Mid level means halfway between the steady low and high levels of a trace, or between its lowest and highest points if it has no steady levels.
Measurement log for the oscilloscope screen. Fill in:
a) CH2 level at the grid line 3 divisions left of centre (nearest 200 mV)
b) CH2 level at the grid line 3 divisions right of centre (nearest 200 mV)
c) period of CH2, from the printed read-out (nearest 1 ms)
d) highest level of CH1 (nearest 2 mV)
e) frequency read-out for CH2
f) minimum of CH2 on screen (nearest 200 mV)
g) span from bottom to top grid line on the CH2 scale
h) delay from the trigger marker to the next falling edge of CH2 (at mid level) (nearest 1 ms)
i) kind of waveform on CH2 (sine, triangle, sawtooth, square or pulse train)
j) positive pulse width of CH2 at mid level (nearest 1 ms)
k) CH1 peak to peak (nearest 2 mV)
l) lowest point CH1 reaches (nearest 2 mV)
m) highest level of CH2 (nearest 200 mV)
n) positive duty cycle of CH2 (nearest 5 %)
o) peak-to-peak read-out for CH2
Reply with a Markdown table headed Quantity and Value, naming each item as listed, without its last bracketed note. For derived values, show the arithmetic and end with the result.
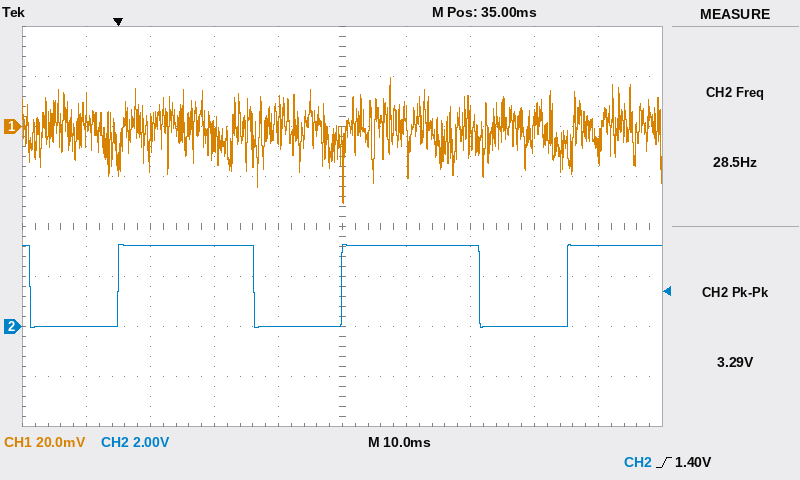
| Quantity | Value |
|---|---|
| CH2 level at the grid line 3 divisions left of centre | 3.2 V |
| CH2 level at the grid line 3 divisions right of centre | 0.0 V |
| period of CH2, from the printed read-out | 1 / 28.5 Hz ≈ 35 ms |
| highest level of CH1 | 20 mV |
| frequency read-out for CH2 | 28.5 Hz |
| minimum of CH2 on screen | 0.0 V |
| span from bottom to top grid line on the CH2 scale | 16 V |
| delay from the trigger marker to the next falling edge of CH2 (at mid level) | 21 ms |
| kind of waveform on CH2 | pulse train |
| positive pulse width of CH2 at mid level | 21 ms |
| CH1 peak to peak | 20 mV − (-30 mV) = 50 mV |
| lowest point CH1 reaches | -30 mV |
| highest level of CH2 | 3.2 V |
| positive duty cycle of CH2 | 60 % |
| peak-to-peak read-out for CH2 | 3.29 V |
